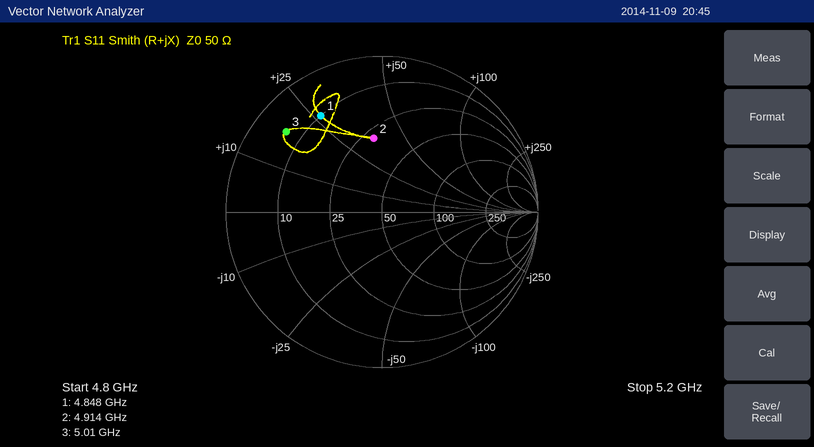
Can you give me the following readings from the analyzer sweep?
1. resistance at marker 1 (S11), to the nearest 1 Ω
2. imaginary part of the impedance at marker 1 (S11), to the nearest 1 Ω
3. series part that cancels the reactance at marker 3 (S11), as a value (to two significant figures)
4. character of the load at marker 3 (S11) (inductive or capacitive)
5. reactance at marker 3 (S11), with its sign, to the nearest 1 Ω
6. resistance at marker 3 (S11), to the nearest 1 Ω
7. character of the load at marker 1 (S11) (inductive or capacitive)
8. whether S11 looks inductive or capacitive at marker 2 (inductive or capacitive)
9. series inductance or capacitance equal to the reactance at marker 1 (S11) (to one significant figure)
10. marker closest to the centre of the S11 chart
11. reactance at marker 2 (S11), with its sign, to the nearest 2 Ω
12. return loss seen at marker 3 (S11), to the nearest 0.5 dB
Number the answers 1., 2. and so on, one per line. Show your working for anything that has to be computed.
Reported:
1. 10 Ω
2. +27 Ω
3. C = 1/(2π × 5.01 GHz × 18 Ω) ≈ 1.8 pF
4. inductive
5. +18 Ω
6. 6 Ω
7. inductive
8. inductive
9. L = 27 Ω/(2π × 4.848 GHz) ≈ 886 pH, so 900 pH to one significant figure
10. marker 2
11. +36 Ω
12. 2.0 dB
